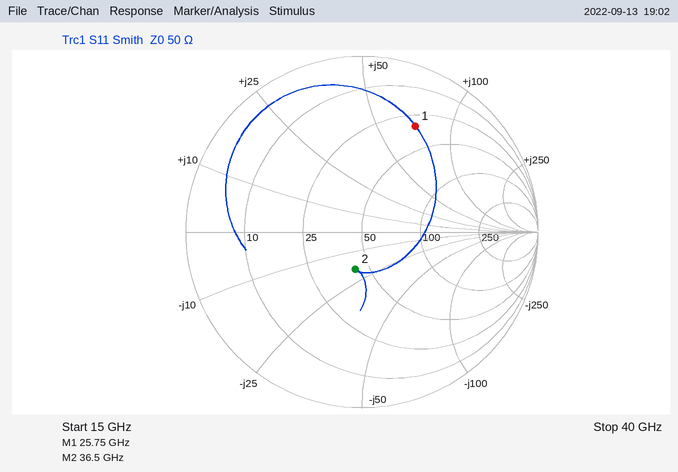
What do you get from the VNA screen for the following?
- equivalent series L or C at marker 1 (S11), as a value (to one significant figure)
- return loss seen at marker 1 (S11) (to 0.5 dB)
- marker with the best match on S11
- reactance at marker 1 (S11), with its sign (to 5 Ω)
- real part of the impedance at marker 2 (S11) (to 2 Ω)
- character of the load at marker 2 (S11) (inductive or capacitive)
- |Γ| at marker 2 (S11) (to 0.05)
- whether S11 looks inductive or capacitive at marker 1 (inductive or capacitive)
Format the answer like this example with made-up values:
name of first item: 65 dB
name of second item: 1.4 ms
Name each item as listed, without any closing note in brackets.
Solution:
equivalent series L or C at marker 1 (S11), as a value: 400 pH
return loss seen at marker 1 (S11): 3.5 dB
marker with the best match on S11: marker 2
reactance at marker 1 (S11), with its sign: +70 Ω
real part of the impedance at marker 2 (S11): 42 Ω
character of the load at marker 2 (S11): capacitive
|Γ| at marker 2 (S11): 0.20
whether S11 looks inductive or capacitive at marker 1: inductive
